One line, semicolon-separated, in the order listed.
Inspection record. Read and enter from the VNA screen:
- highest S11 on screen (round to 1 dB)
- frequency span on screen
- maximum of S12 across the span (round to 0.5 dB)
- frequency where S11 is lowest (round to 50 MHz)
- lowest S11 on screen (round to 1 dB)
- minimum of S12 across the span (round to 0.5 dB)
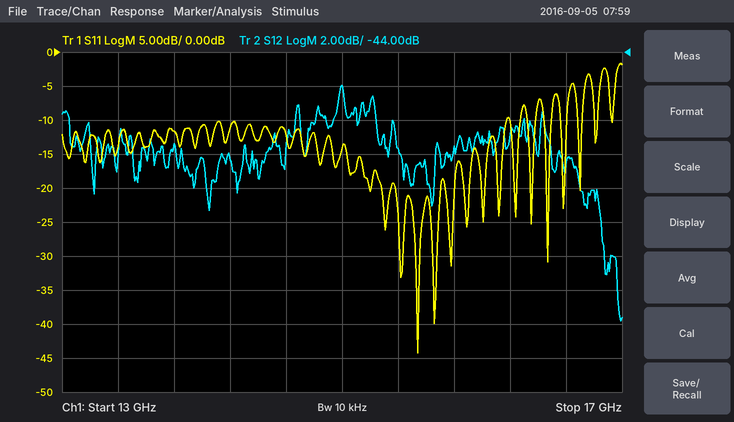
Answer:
-2 dB; 4 GHz; -46.0 dB; 15.55 GHz; -44 dB; -60.0 dB
